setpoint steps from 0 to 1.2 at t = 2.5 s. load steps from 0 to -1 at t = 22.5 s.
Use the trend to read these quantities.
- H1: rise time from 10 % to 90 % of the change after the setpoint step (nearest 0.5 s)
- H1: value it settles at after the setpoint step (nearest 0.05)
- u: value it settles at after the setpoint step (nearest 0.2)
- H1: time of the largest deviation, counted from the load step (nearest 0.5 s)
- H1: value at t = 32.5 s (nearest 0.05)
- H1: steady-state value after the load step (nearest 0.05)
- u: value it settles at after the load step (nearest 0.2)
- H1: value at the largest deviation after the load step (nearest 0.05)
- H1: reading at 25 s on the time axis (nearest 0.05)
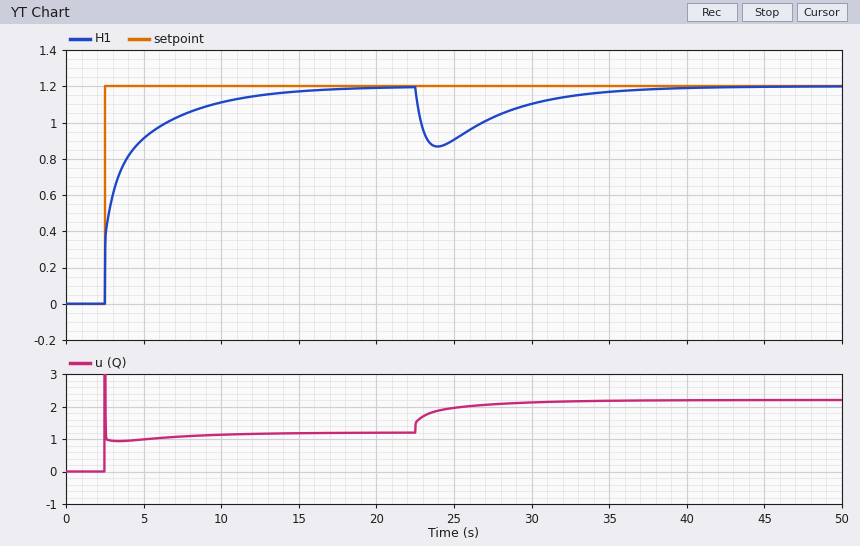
6.0 s
1.20
1.2
1.5 s
1.15
1.20
2.2
0.85
0.90
